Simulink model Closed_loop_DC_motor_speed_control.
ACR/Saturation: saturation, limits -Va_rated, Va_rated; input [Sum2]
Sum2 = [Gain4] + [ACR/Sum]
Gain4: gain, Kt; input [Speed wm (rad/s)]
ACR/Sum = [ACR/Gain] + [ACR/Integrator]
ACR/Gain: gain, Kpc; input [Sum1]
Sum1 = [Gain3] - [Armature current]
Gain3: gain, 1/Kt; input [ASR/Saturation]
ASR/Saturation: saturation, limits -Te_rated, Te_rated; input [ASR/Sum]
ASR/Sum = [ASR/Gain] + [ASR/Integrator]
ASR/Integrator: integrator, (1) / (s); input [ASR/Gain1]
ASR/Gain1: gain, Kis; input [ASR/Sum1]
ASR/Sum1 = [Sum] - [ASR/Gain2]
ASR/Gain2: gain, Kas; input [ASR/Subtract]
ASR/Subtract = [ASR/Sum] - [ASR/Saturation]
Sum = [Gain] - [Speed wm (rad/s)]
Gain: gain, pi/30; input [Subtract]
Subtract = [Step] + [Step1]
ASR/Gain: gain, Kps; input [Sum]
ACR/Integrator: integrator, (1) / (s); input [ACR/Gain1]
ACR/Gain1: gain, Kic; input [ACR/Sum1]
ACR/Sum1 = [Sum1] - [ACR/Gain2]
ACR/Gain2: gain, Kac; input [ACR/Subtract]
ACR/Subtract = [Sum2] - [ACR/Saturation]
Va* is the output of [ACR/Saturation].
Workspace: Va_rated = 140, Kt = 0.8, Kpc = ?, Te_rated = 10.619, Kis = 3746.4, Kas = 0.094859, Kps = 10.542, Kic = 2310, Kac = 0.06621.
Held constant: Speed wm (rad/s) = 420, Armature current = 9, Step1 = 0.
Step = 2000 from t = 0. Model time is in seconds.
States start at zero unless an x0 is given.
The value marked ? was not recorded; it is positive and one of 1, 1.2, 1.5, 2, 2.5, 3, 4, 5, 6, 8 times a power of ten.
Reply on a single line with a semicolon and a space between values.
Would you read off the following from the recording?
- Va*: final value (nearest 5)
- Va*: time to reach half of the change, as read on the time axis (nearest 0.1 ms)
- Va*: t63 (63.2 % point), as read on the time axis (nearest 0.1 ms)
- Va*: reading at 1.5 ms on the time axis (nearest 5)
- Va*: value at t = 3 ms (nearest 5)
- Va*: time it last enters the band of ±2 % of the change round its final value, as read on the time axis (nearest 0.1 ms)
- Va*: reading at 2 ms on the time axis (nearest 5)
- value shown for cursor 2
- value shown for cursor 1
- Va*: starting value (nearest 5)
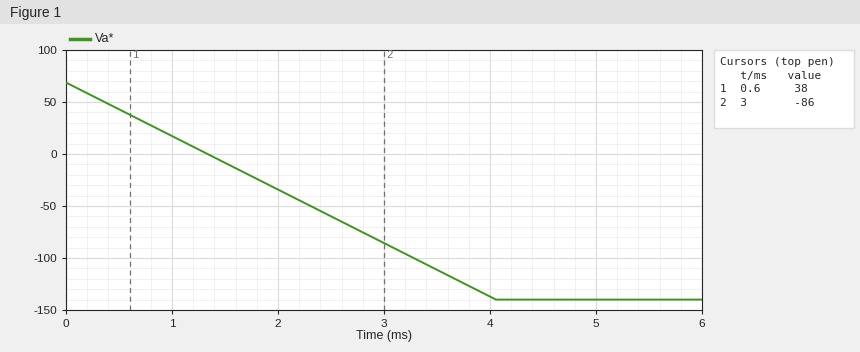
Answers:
-140; 2.0 ms; 2.6 ms; -10; -85; 4.0 ms; -35; -86; 38; 70
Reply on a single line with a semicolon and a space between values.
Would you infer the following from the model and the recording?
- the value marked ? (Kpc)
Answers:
12
